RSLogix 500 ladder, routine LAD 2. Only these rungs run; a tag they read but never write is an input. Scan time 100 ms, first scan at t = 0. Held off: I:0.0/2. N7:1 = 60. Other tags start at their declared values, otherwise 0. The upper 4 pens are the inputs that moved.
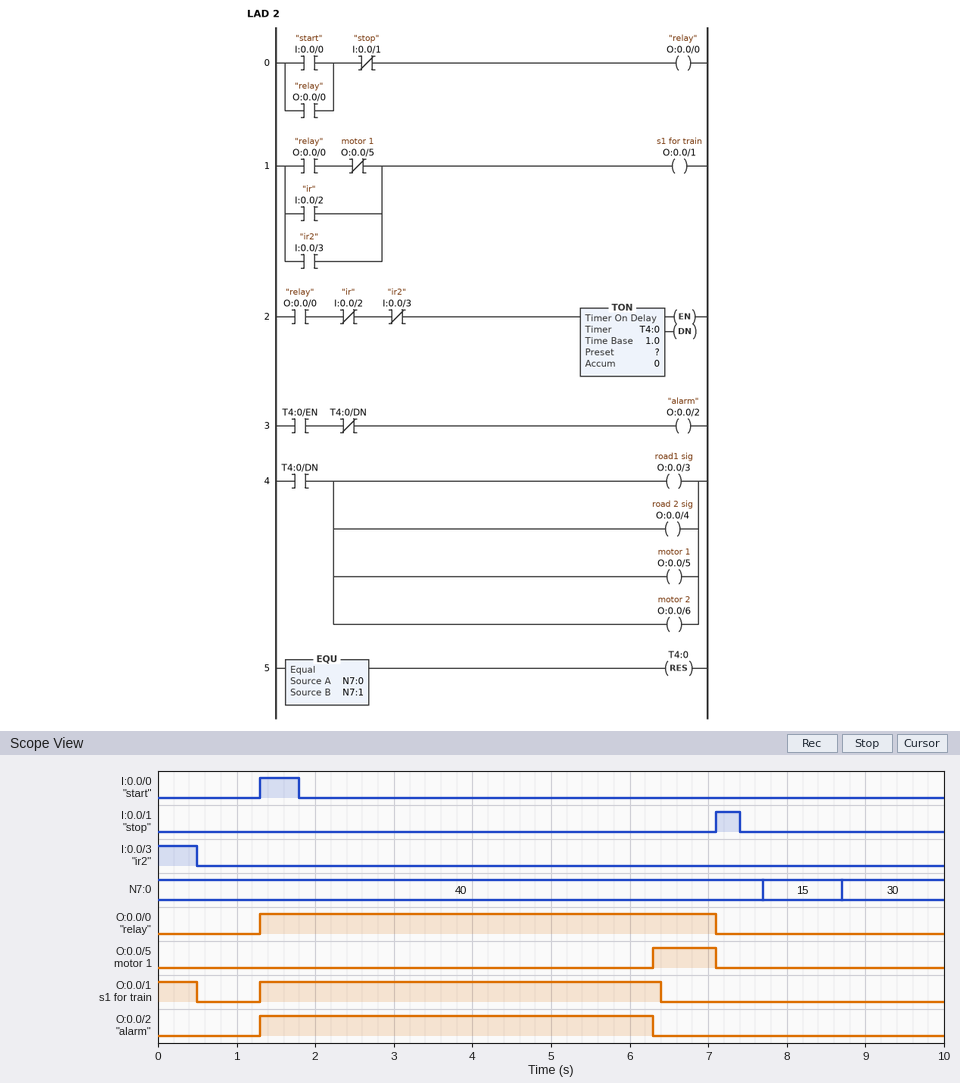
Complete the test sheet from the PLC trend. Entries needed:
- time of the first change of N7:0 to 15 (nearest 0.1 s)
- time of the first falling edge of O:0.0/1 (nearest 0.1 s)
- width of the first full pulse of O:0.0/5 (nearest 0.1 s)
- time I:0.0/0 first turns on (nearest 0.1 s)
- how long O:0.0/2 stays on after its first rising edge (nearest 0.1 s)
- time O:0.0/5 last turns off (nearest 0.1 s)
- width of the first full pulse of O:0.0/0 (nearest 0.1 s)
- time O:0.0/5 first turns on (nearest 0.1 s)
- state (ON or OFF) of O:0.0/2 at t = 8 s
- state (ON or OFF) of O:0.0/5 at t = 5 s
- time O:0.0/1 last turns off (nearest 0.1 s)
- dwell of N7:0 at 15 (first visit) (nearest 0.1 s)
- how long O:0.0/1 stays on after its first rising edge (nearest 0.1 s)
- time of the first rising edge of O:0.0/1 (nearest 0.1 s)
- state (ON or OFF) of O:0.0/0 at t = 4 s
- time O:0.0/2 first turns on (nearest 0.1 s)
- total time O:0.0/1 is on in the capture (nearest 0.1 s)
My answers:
7.7 s
0.5 s
0.8 s
1.3 s
5.0 s
7.1 s
5.8 s
6.3 s
OFF
OFF
6.4 s
1.0 s
5.1 s
1.3 s
ON
1.3 s
5.6 s
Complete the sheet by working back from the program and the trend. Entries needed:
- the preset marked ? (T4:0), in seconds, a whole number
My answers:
5 s
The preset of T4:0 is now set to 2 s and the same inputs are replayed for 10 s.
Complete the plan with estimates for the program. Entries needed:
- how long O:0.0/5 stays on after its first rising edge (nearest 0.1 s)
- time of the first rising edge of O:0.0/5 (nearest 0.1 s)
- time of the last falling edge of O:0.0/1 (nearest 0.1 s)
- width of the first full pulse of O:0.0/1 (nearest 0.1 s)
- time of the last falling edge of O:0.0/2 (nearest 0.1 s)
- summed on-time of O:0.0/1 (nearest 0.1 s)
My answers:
3.8 s
3.3 s
3.4 s
2.1 s
3.3 s
2.6 s
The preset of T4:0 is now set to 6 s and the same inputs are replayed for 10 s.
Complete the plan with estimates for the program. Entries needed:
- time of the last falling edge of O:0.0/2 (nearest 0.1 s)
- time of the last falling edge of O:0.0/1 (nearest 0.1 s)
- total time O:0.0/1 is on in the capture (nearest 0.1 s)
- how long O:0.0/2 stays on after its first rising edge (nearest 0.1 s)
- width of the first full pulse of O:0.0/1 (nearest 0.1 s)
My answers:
7.1 s
7.1 s
6.3 s
5.8 s
5.8 s
